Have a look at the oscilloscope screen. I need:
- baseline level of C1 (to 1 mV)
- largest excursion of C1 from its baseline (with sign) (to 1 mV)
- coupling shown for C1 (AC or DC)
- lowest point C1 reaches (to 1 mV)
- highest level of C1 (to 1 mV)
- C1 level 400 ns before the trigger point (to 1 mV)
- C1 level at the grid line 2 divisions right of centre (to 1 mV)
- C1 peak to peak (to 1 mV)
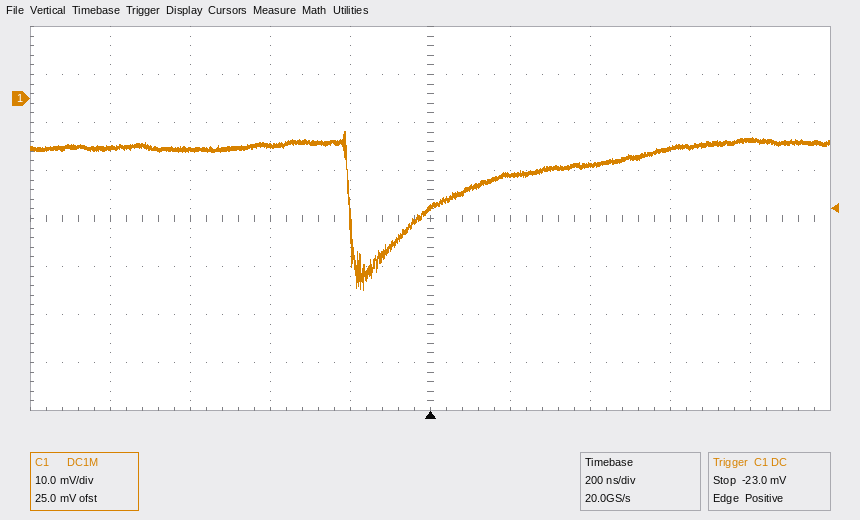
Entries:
-10 mV
-30 mV
DC
-40 mV
-7 mV
-10 mV
-14 mV
33 mV
